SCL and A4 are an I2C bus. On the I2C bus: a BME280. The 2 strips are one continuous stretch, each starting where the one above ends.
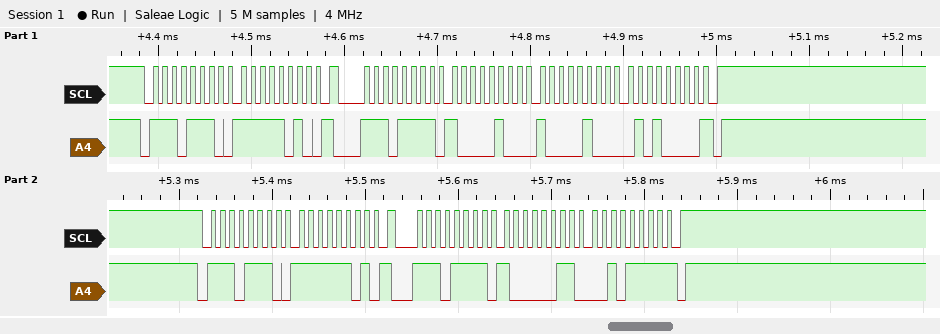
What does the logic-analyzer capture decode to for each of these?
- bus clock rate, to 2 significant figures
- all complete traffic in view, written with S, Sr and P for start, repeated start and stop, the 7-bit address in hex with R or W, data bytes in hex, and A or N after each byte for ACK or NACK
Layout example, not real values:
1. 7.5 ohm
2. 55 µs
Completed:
1. 100 kHz
2. S 77W A FA A Sr 77R A 84 A 84 A 50 N P S 77W A FD A Sr 77R A 83 A 2F N P
